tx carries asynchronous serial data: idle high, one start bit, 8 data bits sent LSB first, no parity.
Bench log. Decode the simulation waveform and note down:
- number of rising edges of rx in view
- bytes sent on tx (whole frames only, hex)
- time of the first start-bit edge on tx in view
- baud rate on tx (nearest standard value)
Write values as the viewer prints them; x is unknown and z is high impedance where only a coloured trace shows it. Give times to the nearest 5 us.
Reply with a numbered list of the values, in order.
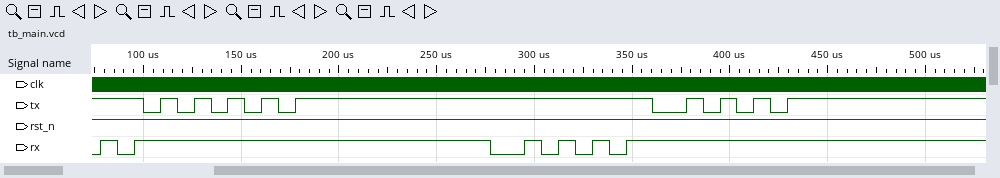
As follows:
1. 6
2. 55, AA
3. 100 us
4. 115200 baud
